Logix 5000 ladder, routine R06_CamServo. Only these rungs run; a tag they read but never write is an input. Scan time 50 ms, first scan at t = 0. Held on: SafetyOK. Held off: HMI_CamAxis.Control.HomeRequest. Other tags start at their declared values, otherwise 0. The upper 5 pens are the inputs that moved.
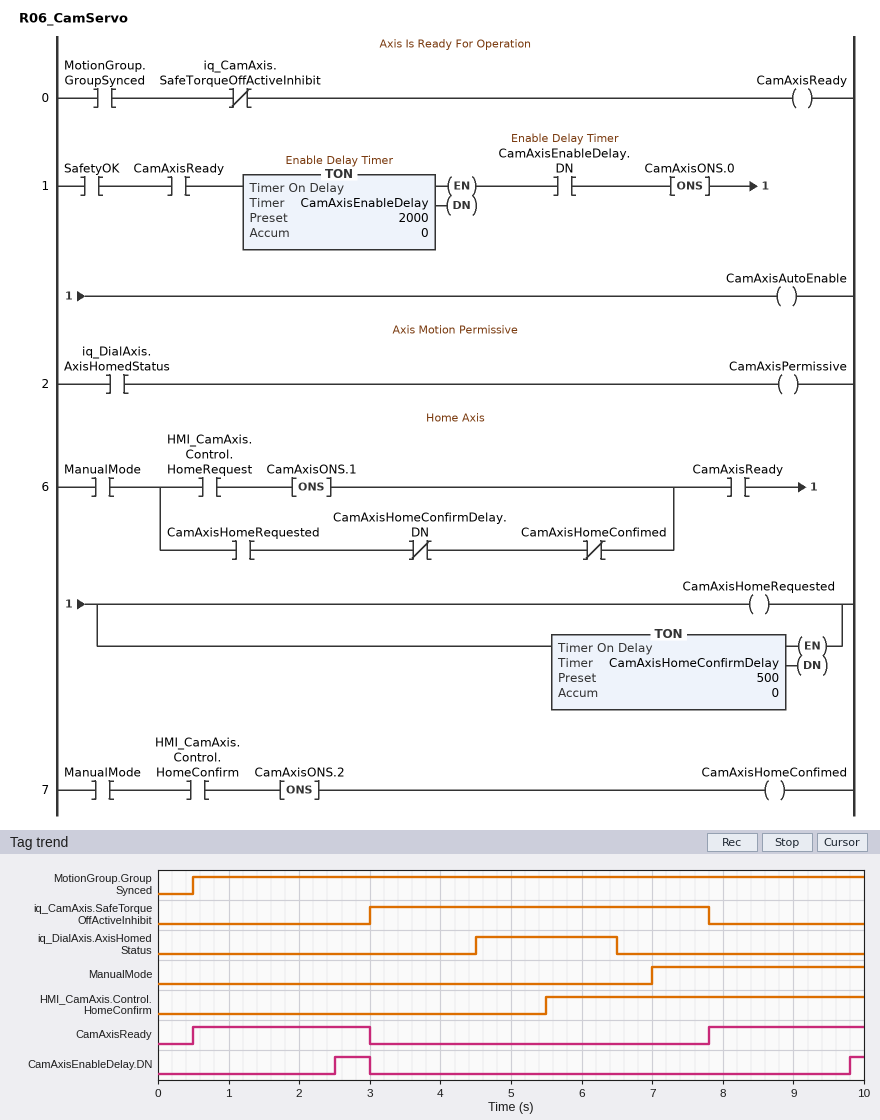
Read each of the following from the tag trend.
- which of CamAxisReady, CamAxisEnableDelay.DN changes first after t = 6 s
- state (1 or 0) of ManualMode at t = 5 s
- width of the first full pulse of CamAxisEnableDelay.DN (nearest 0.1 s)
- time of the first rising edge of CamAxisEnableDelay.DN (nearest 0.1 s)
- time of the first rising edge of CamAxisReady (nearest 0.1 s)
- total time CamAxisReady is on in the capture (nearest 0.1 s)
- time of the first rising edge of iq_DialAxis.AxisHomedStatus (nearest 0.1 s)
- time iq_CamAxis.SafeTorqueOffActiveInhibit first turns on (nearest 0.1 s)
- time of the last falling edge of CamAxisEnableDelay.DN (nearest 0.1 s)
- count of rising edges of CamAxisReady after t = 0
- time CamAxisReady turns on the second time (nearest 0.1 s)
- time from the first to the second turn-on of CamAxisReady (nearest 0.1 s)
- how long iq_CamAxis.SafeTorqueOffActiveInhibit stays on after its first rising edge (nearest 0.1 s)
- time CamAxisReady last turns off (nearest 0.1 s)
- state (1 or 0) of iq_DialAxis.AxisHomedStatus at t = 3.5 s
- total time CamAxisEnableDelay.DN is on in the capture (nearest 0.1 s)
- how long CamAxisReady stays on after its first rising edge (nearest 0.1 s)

CamAxisReady
0
0.5 s
2.5 s
0.5 s
4.7 s
4.5 s
3.0 s
3.0 s
2
7.8 s
7.3 s
4.8 s
3.0 s
0
0.7 s
2.5 s
